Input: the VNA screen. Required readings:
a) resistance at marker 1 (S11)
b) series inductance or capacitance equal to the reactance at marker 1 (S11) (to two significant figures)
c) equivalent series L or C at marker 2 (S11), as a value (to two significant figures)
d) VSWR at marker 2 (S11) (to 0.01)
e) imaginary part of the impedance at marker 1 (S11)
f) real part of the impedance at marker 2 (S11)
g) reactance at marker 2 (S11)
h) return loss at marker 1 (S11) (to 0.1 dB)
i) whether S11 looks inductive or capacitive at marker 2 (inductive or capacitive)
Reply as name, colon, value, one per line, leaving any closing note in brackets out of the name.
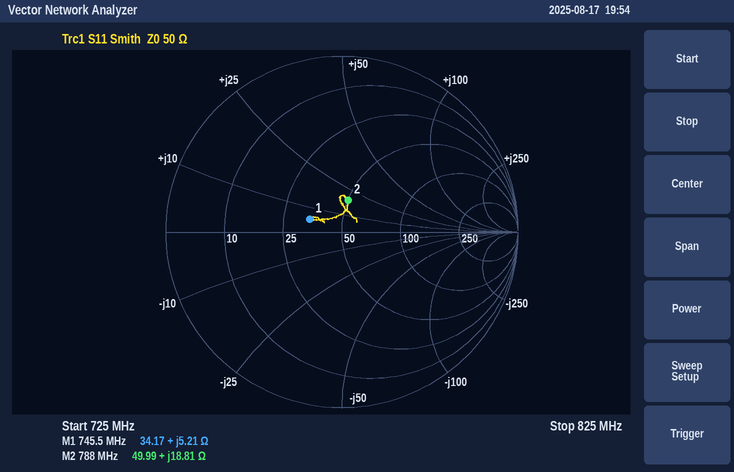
resistance at marker 1: 34.17 Ω
series inductance or capacitance equal to the reactance at marker 1 (S11): 1.1 nH
equivalent series L or C at marker 2 (S11), as a value: 3.8 nH
VSWR at marker 2 (S11): 1.45
imaginary part of the impedance at marker 1: +5.21 Ω
real part of the impedance at marker 2: 49.99 Ω
reactance at marker 2: +18.81 Ω
return loss at marker 1 (S11): 14.1 dB
whether S11 looks inductive or capacitive at marker 2: inductive
